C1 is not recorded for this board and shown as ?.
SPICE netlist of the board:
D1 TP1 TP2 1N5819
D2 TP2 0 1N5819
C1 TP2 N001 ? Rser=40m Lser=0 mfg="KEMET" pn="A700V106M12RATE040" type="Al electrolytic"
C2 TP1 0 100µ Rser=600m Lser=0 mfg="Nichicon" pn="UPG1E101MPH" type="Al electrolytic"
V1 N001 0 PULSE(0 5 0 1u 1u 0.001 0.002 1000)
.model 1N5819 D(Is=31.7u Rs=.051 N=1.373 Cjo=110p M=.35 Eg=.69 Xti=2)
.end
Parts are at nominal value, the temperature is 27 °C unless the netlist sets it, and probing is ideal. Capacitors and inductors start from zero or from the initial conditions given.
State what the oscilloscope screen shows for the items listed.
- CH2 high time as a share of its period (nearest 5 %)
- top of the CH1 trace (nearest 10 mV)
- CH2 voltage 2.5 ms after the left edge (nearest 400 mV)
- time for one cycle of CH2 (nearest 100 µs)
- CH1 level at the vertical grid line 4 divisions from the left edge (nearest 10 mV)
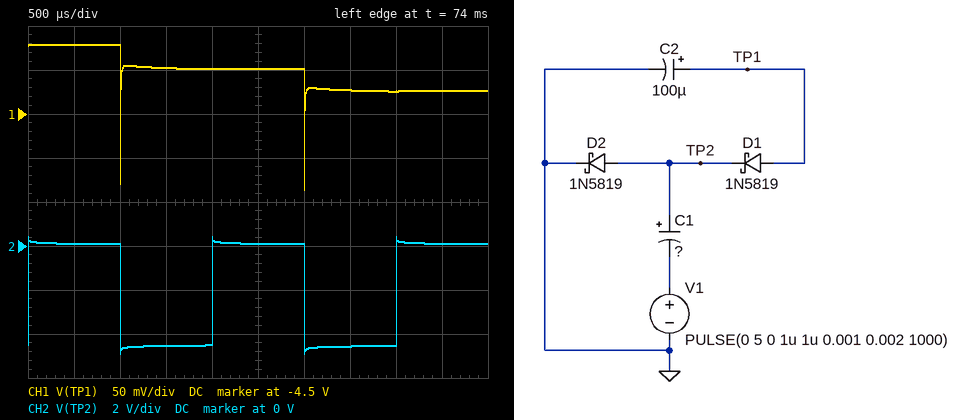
50 %
-4.42 V
0 V
2.0 ms
-4.45 V
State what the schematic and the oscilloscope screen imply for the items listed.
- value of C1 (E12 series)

6.8 µF
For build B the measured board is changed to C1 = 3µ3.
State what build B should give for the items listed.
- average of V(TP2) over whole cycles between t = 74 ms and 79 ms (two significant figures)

-1.7 V
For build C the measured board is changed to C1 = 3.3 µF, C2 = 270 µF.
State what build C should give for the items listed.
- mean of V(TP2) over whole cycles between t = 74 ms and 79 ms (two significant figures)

-920 mV
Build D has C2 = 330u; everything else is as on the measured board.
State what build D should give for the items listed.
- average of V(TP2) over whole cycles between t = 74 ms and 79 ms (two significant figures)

-1.3 V
